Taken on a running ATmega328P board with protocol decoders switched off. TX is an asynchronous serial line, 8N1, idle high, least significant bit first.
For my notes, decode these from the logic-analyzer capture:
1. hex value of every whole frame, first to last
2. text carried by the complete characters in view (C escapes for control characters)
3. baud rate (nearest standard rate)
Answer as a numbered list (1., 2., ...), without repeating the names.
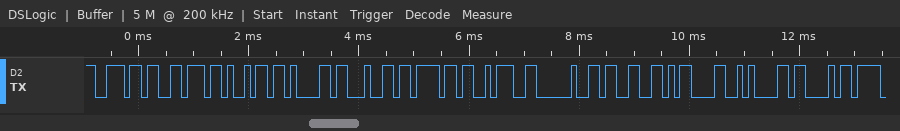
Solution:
1. 0x6E 0x76 0x69 0x61 0x64 0x6F 0x3A 0x20 0x33 0x0D 0x0A 0x43
2. "nviado: 3\r\nC"
3. 9600 baud
